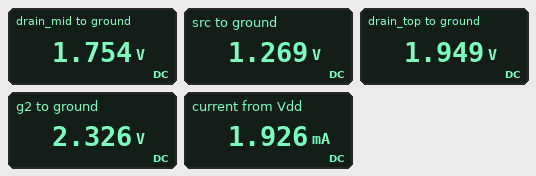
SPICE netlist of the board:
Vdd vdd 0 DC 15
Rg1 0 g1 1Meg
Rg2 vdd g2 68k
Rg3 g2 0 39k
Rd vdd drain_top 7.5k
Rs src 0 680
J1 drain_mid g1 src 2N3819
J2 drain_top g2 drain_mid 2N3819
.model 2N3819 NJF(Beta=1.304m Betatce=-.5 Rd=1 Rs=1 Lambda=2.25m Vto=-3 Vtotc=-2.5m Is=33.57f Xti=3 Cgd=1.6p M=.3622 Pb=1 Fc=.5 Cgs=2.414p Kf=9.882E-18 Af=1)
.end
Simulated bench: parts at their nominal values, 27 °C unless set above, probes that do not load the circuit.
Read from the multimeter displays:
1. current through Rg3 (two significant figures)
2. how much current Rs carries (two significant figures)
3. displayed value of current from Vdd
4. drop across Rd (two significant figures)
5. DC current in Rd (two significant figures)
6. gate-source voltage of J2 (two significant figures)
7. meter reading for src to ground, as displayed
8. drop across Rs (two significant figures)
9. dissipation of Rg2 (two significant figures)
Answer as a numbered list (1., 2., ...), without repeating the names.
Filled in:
1. 60 µA
2. 1.9 mA
3. 1.926 mA
4. 13 V
5. 1.7 mA
6. 570 mV
7. 1.269 V
8. 1.3 V
9. 2.4 mW
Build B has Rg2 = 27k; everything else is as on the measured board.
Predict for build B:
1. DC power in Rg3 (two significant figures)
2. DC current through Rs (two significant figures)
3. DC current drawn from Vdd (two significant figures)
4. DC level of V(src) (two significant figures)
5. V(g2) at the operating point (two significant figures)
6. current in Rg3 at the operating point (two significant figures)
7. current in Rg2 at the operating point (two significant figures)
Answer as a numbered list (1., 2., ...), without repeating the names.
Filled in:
1. 180 µW
2. 2.1 mA
3. 2.2 mA
4. 1.4 V
5. 2.7 V
6. 68 µA
7. 460 µA
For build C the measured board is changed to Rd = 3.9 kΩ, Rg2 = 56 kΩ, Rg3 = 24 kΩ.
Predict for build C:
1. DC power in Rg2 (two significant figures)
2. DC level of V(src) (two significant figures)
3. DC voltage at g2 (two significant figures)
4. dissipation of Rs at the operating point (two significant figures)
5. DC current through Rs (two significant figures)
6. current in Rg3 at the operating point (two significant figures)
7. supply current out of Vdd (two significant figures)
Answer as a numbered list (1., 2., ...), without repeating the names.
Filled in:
1. 2.0 mW
2. 1.6 V
3. 4.5 V
4. 4.0 mW
5. 2.4 mA
6. 190 µA
7. 2.6 mA
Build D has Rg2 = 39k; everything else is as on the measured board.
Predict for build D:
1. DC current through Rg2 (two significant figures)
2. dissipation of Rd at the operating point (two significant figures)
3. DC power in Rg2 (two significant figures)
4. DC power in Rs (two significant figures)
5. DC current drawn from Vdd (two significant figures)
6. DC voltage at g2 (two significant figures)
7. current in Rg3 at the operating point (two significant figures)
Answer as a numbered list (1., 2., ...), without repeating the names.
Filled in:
1. 320 µA
2. 22 mW
3. 4.0 mW
4. 2.7 mW
5. 2.0 mA
6. 2.5 V
7. 64 µA
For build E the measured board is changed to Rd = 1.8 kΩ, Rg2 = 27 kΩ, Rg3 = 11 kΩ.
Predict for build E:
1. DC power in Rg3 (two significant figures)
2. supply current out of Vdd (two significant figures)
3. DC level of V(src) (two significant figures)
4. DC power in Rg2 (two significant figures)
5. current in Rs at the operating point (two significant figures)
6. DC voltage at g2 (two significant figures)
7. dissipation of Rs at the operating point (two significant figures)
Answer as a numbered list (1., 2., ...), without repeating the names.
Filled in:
1. 1.7 mW
2. 2.8 mA
3. 1.6 V
4. 4.2 mW
5. 2.4 mA
6. 4.3 V
7. 4.0 mW
